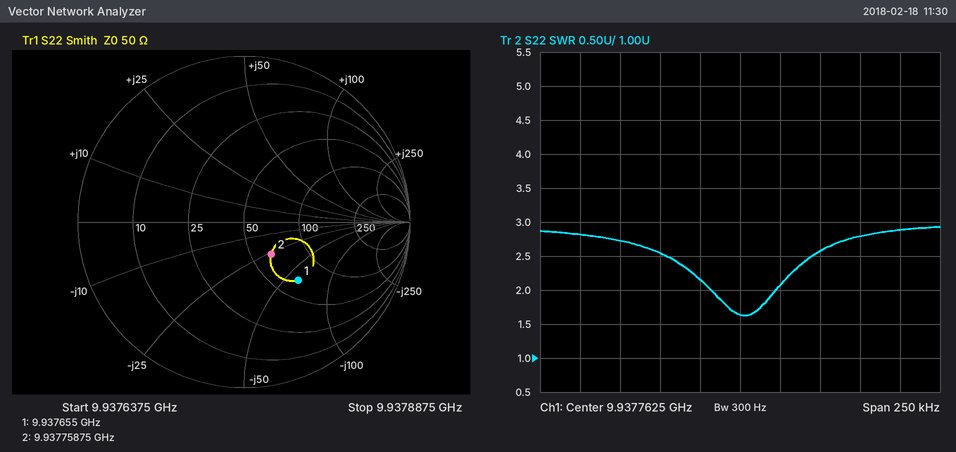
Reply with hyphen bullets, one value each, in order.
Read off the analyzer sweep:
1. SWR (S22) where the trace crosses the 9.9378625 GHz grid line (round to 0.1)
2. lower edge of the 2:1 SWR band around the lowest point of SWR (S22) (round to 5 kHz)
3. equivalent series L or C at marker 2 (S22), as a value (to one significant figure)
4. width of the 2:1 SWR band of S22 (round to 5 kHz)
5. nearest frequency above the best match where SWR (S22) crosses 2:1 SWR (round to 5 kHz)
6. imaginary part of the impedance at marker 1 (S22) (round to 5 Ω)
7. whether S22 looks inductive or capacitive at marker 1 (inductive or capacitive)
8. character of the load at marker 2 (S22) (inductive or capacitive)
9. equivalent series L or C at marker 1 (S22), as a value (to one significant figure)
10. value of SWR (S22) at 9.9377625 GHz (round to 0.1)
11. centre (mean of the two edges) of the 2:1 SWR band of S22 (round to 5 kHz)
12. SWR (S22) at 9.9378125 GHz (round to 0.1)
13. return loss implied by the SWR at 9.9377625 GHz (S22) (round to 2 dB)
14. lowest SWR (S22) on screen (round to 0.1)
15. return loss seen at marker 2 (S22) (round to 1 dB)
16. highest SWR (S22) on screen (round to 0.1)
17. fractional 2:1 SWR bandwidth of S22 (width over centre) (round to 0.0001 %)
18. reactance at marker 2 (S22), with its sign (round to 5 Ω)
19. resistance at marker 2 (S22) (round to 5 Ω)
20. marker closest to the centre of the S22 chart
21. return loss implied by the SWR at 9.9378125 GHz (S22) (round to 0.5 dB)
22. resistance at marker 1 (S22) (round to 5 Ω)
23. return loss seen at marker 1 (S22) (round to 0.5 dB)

- 2.9
- 9.937745 GHz
- 600 fF
- 40 kHz
- 9.937785 GHz
- -60 Ω
- capacitive
- capacitive
- 300 fF
- 1.6
- 9.937765 GHz
- 2.6
- 12 dB
- 1.6
- 12 dB
- 2.9
- 0.0004 %
- -25 Ω
- 65 Ω
- marker 2
- 7.0 dB
- 65 Ω
- 6.5 dB
